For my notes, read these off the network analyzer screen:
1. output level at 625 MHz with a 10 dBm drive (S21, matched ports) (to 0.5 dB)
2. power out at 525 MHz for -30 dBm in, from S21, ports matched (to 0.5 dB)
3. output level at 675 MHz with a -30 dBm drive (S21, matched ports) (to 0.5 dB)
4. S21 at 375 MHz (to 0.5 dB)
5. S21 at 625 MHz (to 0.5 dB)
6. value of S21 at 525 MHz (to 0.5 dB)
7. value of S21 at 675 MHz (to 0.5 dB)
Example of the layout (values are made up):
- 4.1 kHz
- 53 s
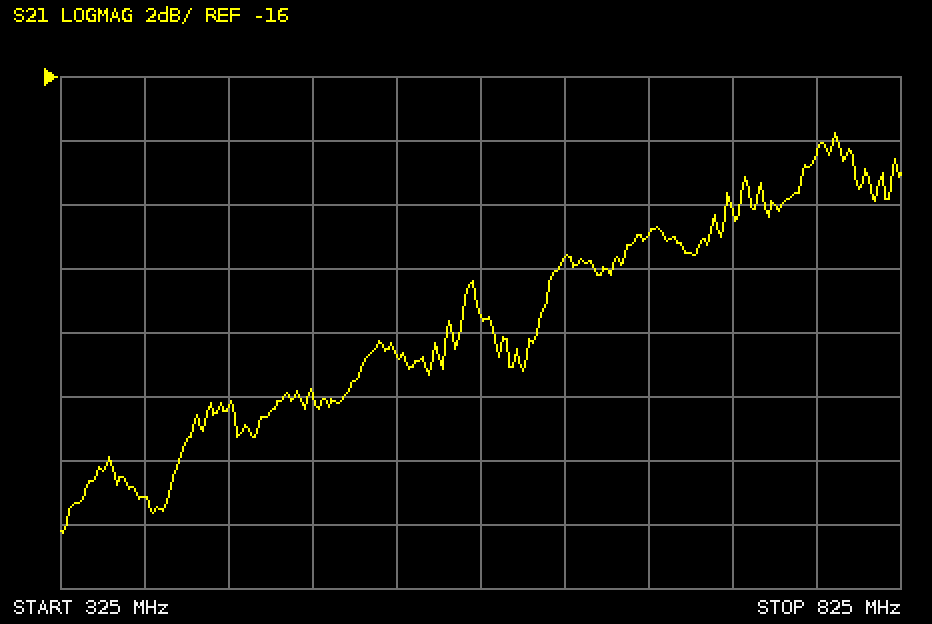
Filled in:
- -11.5 dBm
- -54.5 dBm
- -51.0 dBm
- -29.0 dB
- -21.5 dB
- -24.5 dB
- -21.0 dB
